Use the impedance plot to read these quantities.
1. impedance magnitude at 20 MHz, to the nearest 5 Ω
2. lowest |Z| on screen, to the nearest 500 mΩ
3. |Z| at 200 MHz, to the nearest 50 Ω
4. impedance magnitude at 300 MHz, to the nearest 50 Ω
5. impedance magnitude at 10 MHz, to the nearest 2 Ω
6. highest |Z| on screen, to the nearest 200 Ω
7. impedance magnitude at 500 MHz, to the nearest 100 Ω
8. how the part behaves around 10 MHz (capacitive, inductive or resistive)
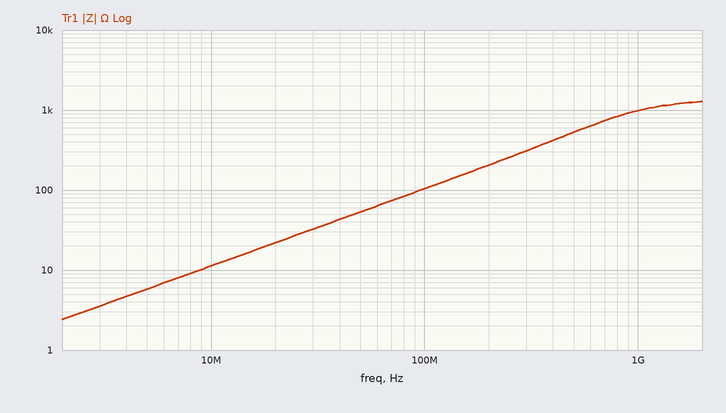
20 Ω
2.5 Ω
200 Ω
300 Ω
12 Ω
1.2 kΩ
500 Ω
inductive
